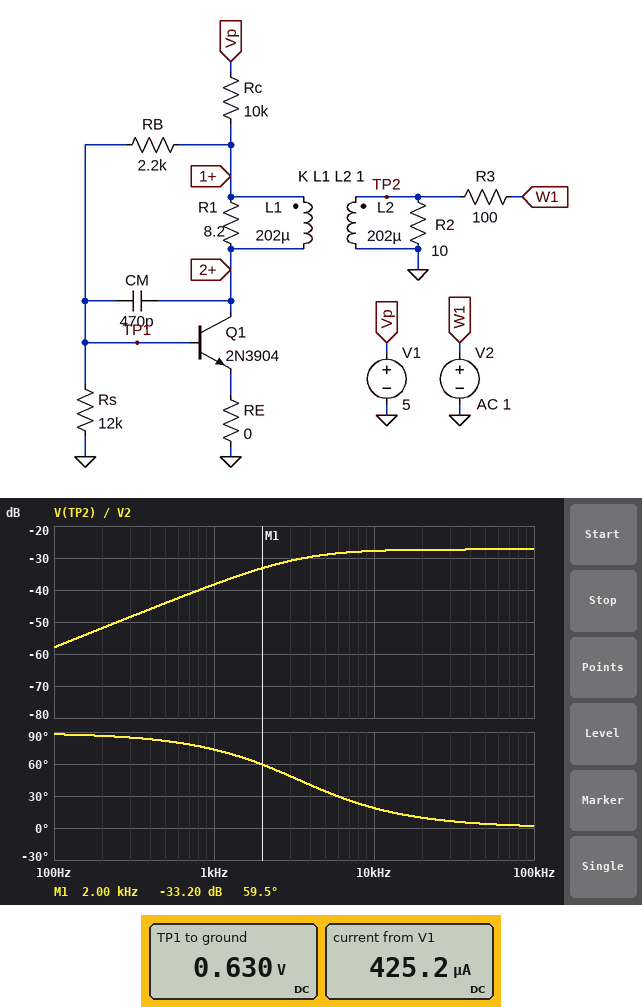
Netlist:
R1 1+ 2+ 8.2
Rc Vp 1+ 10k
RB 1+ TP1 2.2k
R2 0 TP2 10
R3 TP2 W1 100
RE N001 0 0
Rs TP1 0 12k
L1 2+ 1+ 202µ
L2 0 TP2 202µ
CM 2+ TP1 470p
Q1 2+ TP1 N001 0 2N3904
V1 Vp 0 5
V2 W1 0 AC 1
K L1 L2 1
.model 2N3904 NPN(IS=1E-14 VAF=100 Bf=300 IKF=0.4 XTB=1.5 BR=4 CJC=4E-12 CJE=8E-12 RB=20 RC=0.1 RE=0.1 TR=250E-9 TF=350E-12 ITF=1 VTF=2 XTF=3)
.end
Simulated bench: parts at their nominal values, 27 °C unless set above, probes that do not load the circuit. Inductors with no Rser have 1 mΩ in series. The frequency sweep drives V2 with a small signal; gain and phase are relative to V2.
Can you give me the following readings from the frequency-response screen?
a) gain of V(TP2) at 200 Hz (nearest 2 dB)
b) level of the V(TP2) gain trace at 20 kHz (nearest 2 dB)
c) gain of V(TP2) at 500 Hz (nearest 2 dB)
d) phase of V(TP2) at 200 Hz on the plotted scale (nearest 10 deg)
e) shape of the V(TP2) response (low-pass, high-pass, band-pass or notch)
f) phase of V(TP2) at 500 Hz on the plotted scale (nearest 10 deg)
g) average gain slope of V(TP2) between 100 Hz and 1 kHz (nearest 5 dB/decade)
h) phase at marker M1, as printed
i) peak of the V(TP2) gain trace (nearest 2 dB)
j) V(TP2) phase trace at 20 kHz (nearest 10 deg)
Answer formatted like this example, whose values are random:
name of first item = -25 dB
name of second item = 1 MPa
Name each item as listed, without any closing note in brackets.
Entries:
gain of V(TP2) at 200 Hz = -52 dB
level of the V(TP2) gain trace at 20 kHz = -28 dB
gain of V(TP2) at 500 Hz = -44 dB
phase of V(TP2) at 200 Hz on the plotted scale = 90 deg
shape of the V(TP2) response = high-pass
phase of V(TP2) at 500 Hz on the plotted scale = 80 deg
average gain slope of V(TP2) between 100 Hz and 1 kHz = 20 dB/decade
phase at marker M1, as printed = 59.5 deg
peak of the V(TP2) gain trace = -28 dB
V(TP2) phase trace at 20 kHz = 10 deg
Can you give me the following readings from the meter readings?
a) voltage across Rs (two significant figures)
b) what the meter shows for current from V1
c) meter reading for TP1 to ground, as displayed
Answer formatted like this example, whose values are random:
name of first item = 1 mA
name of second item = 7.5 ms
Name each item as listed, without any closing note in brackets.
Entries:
voltage across Rs = 630 mV
what the meter shows for current from V1 = 425.2 µA
meter reading for TP1 to ground, as displayed = 0.630 V
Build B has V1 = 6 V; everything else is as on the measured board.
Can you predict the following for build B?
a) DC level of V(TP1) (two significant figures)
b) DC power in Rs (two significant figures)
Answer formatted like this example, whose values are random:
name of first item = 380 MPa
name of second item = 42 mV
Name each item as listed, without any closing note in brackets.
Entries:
DC level of V(TP1) = 640 mV
DC power in Rs = 34 µW
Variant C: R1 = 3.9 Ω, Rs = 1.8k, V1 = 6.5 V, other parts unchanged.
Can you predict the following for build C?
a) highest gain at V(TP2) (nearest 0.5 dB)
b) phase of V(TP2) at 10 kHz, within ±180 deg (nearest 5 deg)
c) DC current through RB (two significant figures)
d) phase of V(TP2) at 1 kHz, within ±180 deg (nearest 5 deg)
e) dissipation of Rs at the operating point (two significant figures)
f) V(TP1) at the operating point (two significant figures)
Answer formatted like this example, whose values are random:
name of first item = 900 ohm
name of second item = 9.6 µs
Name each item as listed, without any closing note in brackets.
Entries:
highest gain at V(TP2) = -31.5 dB
phase of V(TP2) at 10 kHz, within ±180 deg = 10 deg
DC current through RB = 340 µA
phase of V(TP2) at 1 kHz, within ±180 deg = 65 deg
dissipation of Rs at the operating point = 210 µW
V(TP1) at the operating point = 610 mV
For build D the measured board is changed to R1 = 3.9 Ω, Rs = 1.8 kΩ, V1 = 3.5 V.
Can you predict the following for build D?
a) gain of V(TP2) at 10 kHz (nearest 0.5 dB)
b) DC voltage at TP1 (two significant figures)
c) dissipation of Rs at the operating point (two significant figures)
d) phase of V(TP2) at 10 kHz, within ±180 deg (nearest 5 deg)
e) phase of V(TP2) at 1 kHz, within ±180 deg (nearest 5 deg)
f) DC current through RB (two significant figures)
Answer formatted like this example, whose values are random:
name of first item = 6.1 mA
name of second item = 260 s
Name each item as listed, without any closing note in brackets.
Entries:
gain of V(TP2) at 10 kHz = -31.5 dB
DC voltage at TP1 = 450 mV
dissipation of Rs at the operating point = 110 µW
phase of V(TP2) at 10 kHz, within ±180 deg = 10 deg
phase of V(TP2) at 1 kHz, within ±180 deg = 65 deg
DC current through RB = 250 µA
